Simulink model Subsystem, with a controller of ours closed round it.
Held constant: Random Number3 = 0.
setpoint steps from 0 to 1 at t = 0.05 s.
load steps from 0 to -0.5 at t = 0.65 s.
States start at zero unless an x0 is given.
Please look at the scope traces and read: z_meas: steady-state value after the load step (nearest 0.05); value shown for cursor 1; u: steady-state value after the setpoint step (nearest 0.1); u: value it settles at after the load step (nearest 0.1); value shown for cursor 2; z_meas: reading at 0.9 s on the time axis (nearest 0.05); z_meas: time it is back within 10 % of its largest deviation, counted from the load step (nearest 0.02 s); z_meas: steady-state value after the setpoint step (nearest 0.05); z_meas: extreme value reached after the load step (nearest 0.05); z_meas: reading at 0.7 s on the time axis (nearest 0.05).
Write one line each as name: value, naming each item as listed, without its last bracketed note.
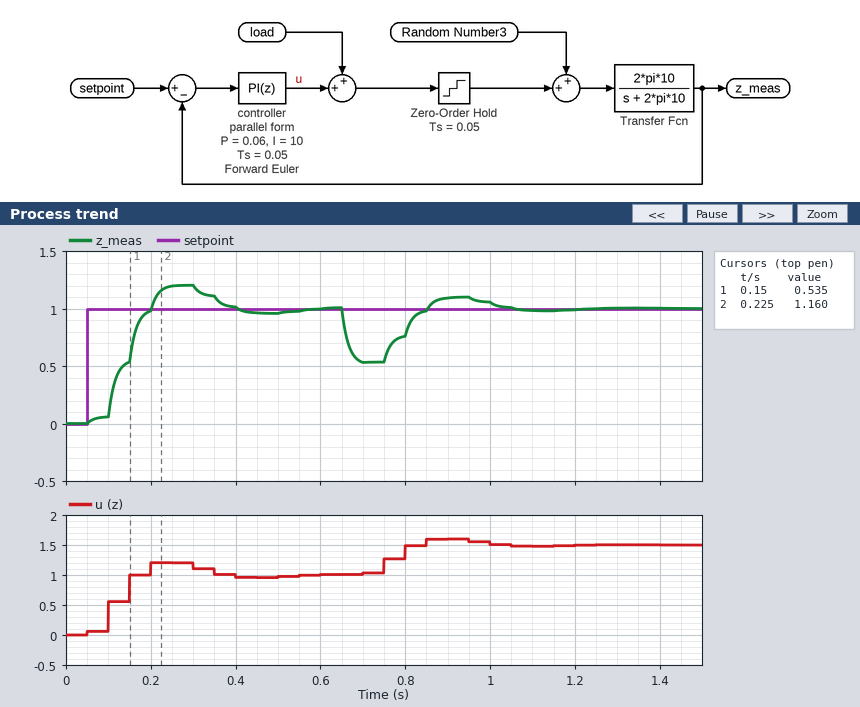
z_meas: steady-state value after the load step: 1.00
value shown for cursor 1: 0.535
u: steady-state value after the setpoint step: 1.0
u: value it settles at after the load step: 1.5
value shown for cursor 2: 1.160
z_meas: reading at 0.9 s on the time axis: 1.10
z_meas: time it is back within 10 % of its largest deviation, counted from the load step: 0.36 s
z_meas: steady-state value after the setpoint step: 1.00
z_meas: extreme value reached after the load step: 0.55
z_meas: reading at 0.7 s on the time axis: 0.55
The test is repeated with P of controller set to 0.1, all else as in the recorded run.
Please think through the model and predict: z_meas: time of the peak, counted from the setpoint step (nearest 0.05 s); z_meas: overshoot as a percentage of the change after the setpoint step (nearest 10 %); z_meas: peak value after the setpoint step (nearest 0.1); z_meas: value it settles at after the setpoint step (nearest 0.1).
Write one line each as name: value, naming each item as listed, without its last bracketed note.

z_meas: time of the peak, counted from the setpoint step: 0.25 s
z_meas: overshoot as a percentage of the change after the setpoint step: 20 %
z_meas: peak value after the setpoint step: 1.2
z_meas: value it settles at after the setpoint step: 1.0
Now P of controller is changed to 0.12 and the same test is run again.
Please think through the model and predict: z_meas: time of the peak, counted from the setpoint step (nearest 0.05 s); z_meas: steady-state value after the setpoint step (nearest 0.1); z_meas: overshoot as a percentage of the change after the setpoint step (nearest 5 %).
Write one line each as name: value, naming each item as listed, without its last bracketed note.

z_meas: time of the peak, counted from the setpoint step: 0.20 s
z_meas: steady-state value after the setpoint step: 1.0
z_meas: overshoot as a percentage of the change after the setpoint step: 15 %
